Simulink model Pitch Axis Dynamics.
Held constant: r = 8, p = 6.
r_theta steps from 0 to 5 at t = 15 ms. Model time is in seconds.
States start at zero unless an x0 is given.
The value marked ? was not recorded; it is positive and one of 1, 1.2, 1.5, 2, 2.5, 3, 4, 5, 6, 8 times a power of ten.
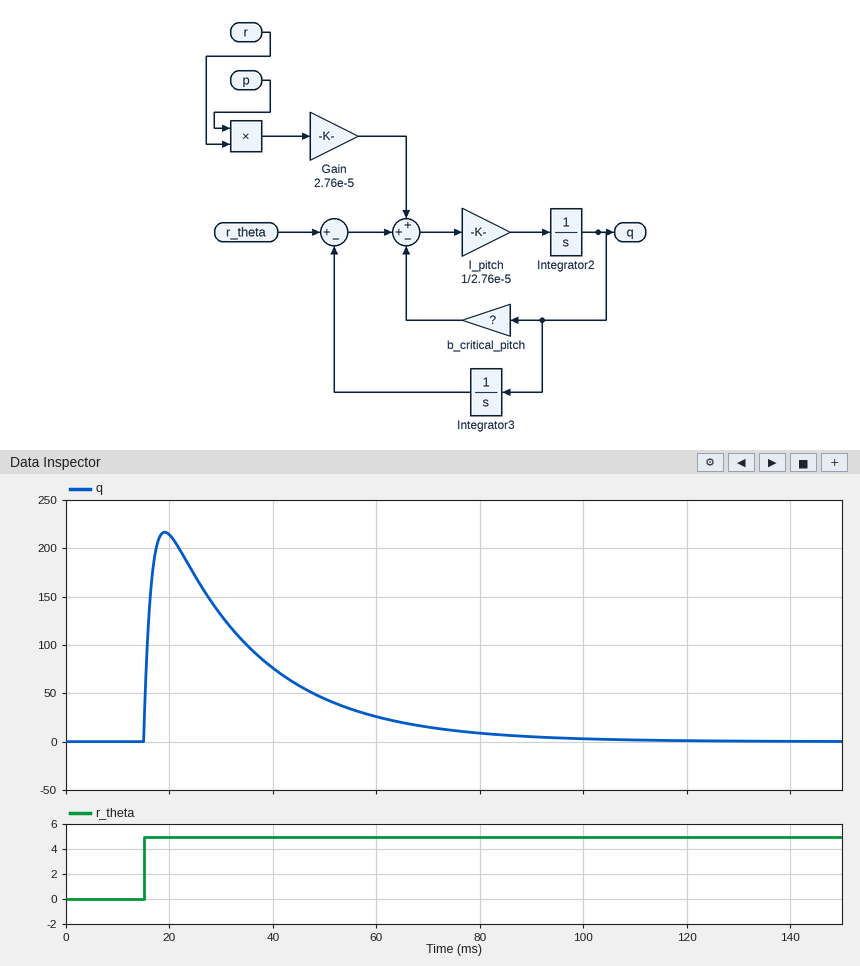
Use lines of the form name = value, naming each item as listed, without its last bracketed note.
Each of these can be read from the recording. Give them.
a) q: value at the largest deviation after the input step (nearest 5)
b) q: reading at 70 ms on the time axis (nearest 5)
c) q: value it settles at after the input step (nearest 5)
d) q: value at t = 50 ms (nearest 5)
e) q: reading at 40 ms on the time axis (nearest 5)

q: value at the largest deviation after the input step = 215
q: reading at 70 ms on the time axis = 15
q: value it settles at after the input step = 0
q: value at t = 50 ms = 45
q: reading at 40 ms on the time axis = 75
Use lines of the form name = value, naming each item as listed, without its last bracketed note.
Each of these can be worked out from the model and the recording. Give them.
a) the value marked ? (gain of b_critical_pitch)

the value marked ? = 0.02
